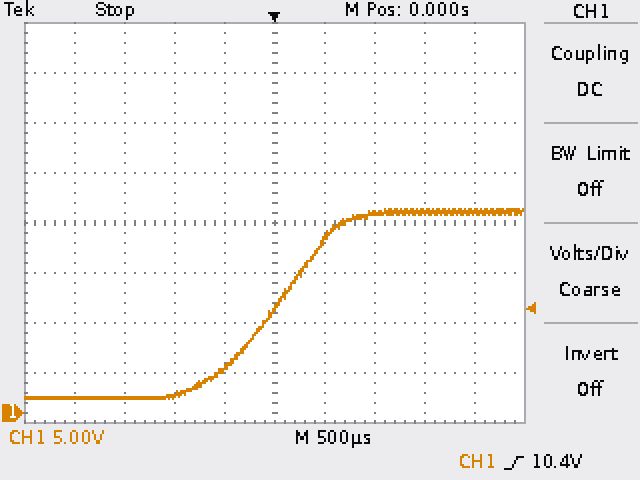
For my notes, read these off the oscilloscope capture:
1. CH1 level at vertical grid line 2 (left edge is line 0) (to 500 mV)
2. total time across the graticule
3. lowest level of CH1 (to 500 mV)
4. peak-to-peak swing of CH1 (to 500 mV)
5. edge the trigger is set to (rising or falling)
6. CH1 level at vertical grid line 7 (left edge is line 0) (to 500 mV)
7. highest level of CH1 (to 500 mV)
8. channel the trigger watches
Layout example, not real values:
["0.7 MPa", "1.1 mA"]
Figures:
["1.5 V", "5 ms", "1.5 V", "19.0 V", "rising", "20.0 V", "20.5 V", "CH1"]
